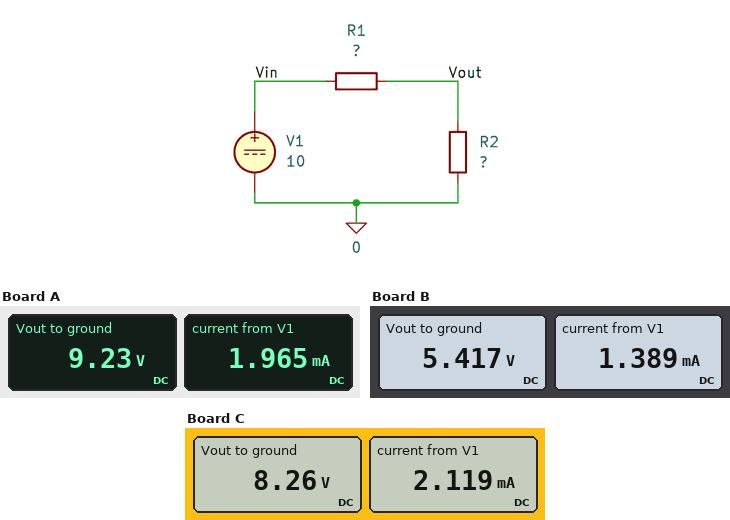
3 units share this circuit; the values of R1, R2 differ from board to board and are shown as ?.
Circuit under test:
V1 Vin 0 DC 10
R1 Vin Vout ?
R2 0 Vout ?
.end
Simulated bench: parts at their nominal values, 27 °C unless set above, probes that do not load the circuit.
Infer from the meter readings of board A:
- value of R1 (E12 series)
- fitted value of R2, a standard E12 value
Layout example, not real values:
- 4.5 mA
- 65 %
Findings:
- 390 Ω
- 4.7 kΩ
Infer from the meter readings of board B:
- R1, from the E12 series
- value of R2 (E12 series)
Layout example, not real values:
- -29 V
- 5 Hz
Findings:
- 3.3 kΩ
- 3.9 kΩ
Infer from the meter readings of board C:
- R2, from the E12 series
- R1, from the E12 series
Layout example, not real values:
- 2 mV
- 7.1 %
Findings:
- 3.9 kΩ
- 820 Ω
